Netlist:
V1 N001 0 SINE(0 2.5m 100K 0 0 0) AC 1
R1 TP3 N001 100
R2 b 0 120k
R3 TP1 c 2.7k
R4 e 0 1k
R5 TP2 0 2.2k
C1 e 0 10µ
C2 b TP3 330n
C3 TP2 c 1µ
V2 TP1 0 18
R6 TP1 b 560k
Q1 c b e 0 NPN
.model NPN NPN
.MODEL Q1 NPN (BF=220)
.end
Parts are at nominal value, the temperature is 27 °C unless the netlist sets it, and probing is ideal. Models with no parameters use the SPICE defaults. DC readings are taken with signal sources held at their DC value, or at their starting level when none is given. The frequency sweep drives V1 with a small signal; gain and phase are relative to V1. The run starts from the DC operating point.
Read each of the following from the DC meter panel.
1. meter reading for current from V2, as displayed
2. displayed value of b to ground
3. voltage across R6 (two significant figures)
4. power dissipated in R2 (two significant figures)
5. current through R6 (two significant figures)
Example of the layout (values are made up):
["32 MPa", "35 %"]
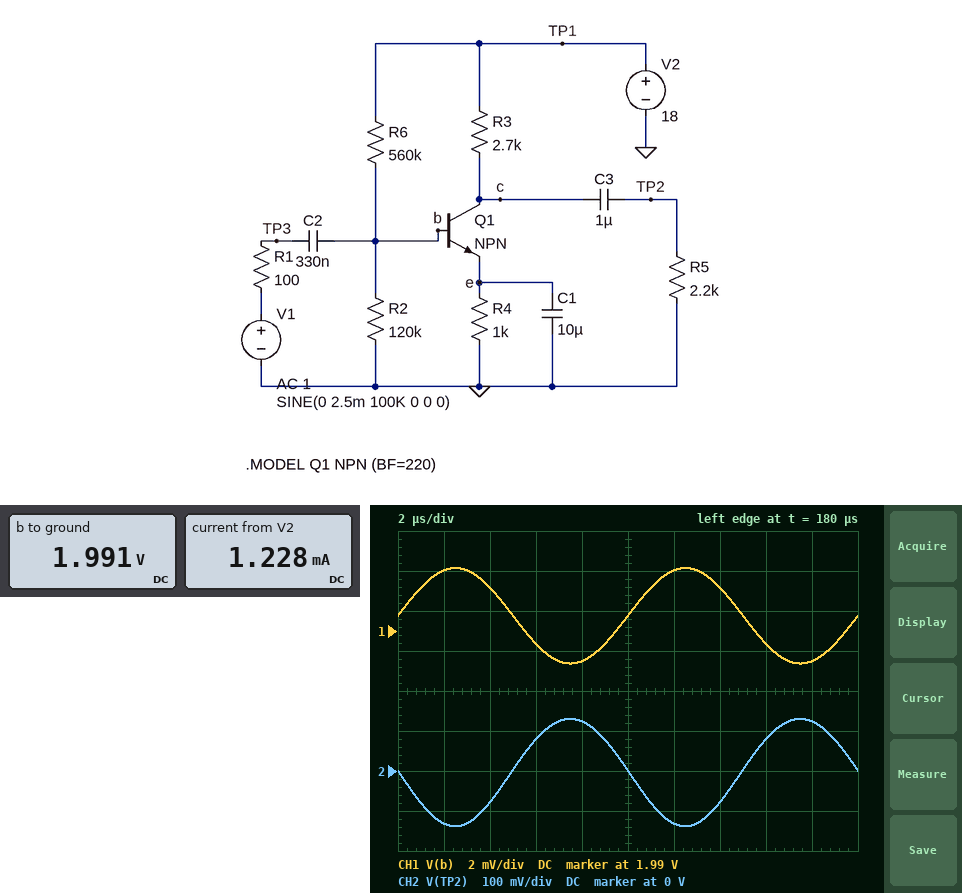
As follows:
["1.228 mA", "1.991 V", "16 V", "33 µW", "29 µA"]
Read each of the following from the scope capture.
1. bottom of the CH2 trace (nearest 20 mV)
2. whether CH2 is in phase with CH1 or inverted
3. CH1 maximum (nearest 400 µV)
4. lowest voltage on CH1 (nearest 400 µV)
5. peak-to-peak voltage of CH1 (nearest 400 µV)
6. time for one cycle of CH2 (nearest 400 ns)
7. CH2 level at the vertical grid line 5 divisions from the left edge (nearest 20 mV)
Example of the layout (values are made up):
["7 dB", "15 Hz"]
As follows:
["-140 mV", "inverted", "1.9932 V", "1.9884 V", "4.8 mV", "10.0 µs", "0 V"]
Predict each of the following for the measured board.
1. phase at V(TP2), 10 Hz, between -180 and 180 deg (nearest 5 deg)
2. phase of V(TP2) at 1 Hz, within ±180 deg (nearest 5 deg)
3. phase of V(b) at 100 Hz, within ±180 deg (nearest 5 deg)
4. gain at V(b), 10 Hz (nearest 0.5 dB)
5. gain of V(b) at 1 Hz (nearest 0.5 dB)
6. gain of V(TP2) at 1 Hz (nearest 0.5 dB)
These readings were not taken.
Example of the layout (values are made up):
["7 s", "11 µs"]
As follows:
["-40 deg", "-5 deg", "5 deg", "-4.0 dB", "-19.5 dB", "-48.5 dB"]
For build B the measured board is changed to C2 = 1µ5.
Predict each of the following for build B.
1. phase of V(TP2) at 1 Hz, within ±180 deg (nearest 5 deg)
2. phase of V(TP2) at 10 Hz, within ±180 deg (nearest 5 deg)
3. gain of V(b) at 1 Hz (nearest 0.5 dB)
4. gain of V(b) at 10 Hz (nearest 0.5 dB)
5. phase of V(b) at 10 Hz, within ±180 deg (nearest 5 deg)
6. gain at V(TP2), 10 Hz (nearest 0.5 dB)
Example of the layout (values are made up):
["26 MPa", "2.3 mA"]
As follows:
["-25 deg", "-65 deg", "-7.5 dB", "-0.5 dB", "10 deg", "-8.5 dB"]
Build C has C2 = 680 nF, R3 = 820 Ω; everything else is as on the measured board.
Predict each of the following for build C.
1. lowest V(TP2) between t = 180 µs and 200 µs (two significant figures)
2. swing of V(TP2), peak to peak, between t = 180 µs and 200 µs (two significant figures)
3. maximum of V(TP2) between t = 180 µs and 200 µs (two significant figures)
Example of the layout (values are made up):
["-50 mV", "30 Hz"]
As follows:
["-68 mV", "130 mV", "64 mV"]
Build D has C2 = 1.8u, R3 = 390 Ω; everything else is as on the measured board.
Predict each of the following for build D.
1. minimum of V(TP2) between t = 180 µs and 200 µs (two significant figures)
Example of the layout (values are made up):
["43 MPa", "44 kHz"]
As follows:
["-38 mV"]
